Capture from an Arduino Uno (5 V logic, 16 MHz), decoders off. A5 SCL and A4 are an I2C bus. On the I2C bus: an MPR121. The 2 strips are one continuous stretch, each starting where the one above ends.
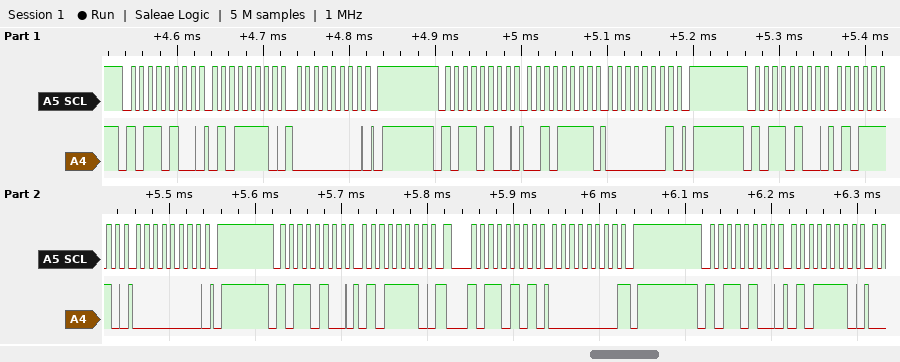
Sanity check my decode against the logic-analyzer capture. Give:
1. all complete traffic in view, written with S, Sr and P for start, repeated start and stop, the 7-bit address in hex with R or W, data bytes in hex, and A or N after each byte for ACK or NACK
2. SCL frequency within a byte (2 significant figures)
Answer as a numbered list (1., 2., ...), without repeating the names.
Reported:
1. S 5AW A 5E A 00 A P S 5AW A 2F A 01 A P S 5AW A 5E A 00 A P S 5AW A 5E A Sr 5AR A 00 N P S 5AW A 5E A
2. 100 kHz
